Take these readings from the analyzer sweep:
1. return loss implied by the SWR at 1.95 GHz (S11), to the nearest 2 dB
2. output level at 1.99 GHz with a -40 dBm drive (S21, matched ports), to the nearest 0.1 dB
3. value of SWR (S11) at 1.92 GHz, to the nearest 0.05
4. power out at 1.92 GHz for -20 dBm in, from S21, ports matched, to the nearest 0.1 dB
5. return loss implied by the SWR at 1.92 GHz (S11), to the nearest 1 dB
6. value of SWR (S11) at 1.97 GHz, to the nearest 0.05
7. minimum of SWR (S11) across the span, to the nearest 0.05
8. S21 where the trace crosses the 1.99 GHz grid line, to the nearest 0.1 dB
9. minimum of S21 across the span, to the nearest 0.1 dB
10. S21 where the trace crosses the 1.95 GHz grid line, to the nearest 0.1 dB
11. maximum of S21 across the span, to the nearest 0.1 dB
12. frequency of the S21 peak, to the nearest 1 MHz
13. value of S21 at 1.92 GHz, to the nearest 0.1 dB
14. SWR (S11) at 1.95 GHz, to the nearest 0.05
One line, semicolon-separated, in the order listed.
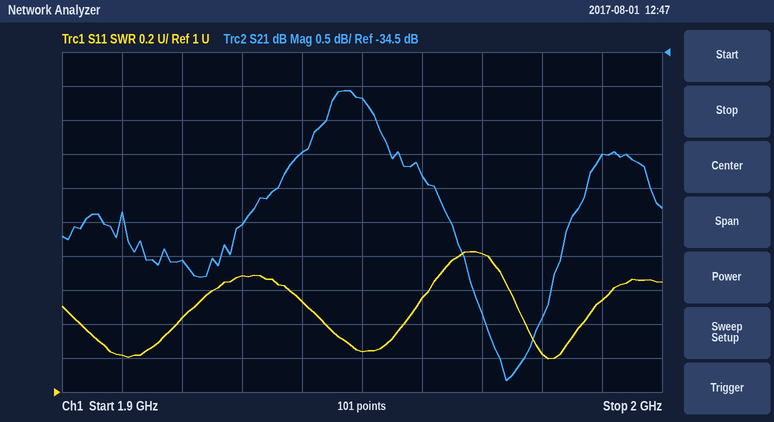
20 dB; -76.0 dBm; 1.45; -57.6 dBm; 15 dB; 1.80; 1.20; -36.0 dB; -39.3 dB; -35.2 dB; -35.1 dB; 1.947 GHz; -37.6 dB; 1.25
